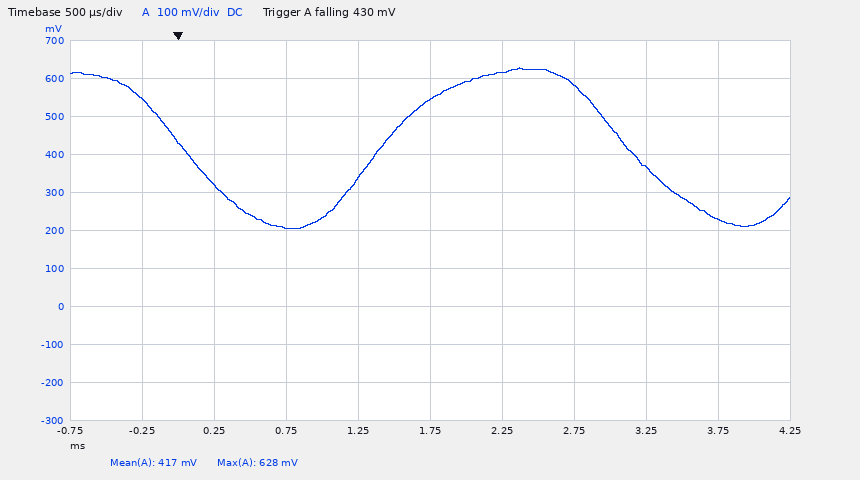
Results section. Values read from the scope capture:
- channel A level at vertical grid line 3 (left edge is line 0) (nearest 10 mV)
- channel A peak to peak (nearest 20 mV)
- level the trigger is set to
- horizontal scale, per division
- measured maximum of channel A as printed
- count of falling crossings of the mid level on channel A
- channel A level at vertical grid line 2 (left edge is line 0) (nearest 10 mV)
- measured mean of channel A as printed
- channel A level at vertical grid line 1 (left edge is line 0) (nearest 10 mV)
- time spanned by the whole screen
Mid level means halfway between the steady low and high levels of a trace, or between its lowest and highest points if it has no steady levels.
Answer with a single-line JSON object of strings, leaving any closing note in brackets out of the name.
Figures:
{"channel A level at vertical grid line 3 (left edge is line 0)": "210 mV", "channel A peak to peak": "420 mV", "level the trigger is set to": "430 mV", "horizontal scale, per division": "500 µs", "measured maximum of channel A as printed": "628 mV", "count of falling crossings of the mid level on channel A": "2", "channel A level at vertical grid line 2 (left edge is line 0)": "320 mV", "measured mean of channel A as printed": "417 mV", "channel A level at vertical grid line 1 (left edge is line 0)": "550 mV", "time spanned by the whole screen": "5 ms"}
